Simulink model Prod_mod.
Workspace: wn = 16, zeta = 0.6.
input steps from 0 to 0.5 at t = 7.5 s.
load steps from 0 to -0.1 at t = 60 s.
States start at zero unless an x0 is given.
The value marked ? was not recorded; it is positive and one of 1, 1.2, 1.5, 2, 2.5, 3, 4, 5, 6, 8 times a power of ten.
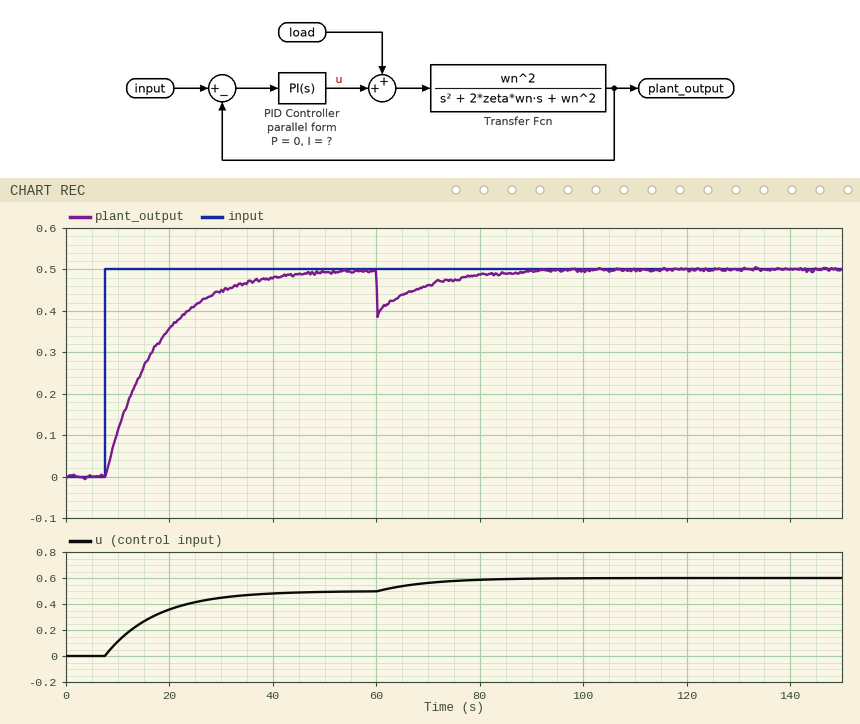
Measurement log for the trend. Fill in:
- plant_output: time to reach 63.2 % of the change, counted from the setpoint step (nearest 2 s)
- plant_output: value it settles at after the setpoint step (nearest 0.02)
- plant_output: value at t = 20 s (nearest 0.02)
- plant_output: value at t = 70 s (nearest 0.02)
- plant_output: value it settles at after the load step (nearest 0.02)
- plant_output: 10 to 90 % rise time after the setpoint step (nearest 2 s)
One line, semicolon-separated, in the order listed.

10 s; 0.50; 0.36; 0.46; 0.50; 22 s
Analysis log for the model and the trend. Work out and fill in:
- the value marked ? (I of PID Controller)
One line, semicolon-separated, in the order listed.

0.1
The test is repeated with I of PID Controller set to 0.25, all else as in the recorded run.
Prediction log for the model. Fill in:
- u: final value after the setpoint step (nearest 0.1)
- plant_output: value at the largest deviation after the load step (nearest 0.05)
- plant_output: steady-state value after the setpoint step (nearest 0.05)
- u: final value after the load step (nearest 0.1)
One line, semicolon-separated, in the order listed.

0.5; 0.40; 0.50; 0.6
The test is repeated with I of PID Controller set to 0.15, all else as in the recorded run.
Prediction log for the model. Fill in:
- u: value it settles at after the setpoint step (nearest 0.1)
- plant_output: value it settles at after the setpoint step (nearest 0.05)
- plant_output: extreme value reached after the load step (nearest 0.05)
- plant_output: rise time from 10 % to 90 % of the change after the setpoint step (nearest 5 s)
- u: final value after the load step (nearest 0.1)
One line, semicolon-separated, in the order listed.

0.5; 0.50; 0.40; 15 s; 0.6
